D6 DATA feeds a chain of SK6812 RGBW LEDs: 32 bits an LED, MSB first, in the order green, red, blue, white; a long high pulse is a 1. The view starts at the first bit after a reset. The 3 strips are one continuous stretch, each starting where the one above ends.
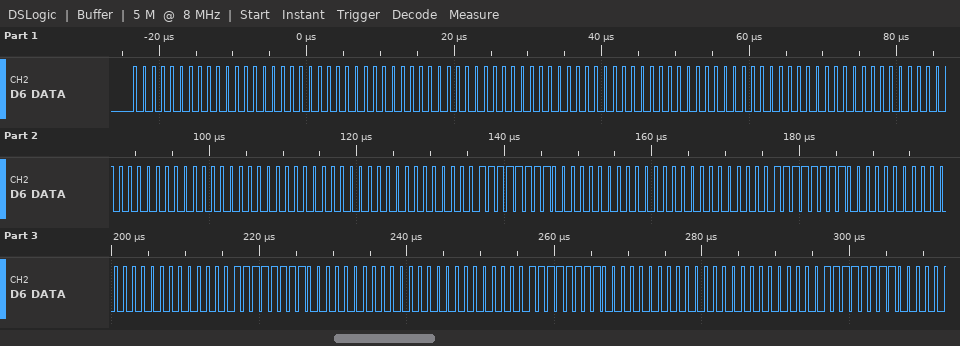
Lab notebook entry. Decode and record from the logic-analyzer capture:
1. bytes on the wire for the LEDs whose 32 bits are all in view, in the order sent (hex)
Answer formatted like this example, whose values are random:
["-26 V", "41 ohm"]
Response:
["00 00 00 00 00 00 00 00 00 00 00 00 00 00 00 00 FF 00 00 00 FF 00 00 00 FF 00 00 00 FF 00 00 00"]
